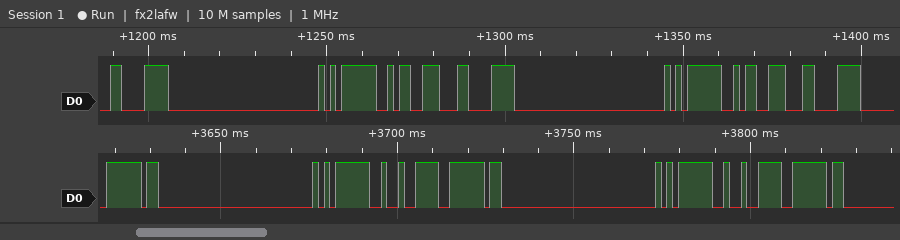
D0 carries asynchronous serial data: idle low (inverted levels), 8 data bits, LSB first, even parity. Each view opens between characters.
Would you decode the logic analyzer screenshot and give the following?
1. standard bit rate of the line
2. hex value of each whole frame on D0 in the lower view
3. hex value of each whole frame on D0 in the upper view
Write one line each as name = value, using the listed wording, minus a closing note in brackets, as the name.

standard bit rate of the line = 600 baud
hex value of each whole frame on D0 in the lower view = 20, 05, 1B, 20, 05, 1B, 20
hex value of each whole frame on D0 in the upper view = 1E, 05, 19, 1E, 05, 19, 1E
